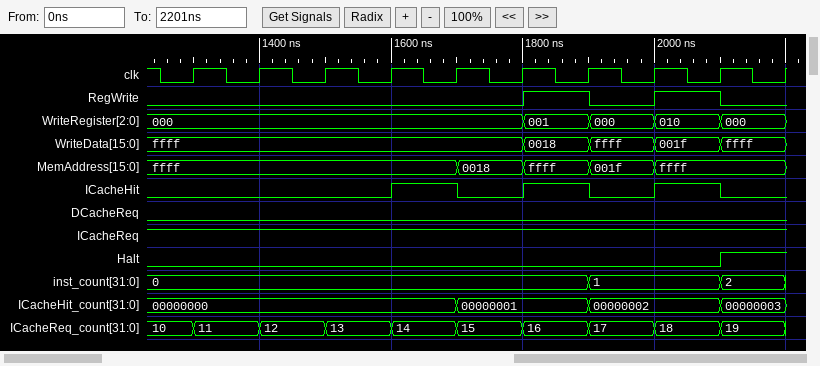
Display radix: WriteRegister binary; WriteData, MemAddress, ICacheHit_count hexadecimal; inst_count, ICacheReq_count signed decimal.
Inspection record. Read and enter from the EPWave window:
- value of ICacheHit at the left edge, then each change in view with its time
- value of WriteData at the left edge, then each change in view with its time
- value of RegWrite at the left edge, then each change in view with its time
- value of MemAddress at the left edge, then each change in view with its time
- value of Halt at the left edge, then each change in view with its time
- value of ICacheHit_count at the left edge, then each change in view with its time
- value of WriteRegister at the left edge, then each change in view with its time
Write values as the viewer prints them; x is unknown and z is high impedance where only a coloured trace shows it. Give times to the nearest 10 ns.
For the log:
0, 1 at 1600 ns, 0 at 1700 ns, 1 at 1800 ns, 0 at 1900 ns, 1 at 2000 ns, 0 at 2100 ns
ffff, 0018 at 1800 ns, ffff at 1900 ns, 001f at 2000 ns, ffff at 2100 ns
0, 1 at 1800 ns, 0 at 1900 ns, 1 at 2000 ns, 0 at 2100 ns
ffff, 0018 at 1700 ns, ffff at 1800 ns, 001f at 1900 ns, ffff at 2000 ns
0, 1 at 2100 ns
00000000, 00000001 at 1700 ns, 00000002 at 1900 ns, 00000003 at 2100 ns
000, 001 at 1800 ns, 000 at 1900 ns, 010 at 2000 ns, 000 at 2100 ns
